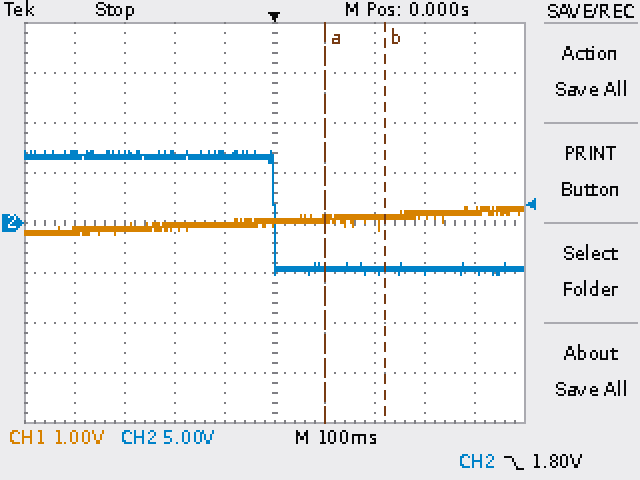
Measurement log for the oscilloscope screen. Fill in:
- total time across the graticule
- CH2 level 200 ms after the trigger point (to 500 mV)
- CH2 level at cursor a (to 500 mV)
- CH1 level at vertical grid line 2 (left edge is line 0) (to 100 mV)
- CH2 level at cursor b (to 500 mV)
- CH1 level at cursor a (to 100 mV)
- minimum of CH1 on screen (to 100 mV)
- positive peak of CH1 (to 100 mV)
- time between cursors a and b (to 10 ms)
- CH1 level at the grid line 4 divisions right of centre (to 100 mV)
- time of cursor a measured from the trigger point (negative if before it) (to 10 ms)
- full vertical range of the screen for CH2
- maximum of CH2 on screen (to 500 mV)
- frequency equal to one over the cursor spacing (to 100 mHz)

1 s
-4.5 V
-4.5 V
-100 mV
-5.0 V
100 mV
-200 mV
300 mV
120 ms
200 mV
+100 ms
40 V
7.0 V
8.3 Hz
